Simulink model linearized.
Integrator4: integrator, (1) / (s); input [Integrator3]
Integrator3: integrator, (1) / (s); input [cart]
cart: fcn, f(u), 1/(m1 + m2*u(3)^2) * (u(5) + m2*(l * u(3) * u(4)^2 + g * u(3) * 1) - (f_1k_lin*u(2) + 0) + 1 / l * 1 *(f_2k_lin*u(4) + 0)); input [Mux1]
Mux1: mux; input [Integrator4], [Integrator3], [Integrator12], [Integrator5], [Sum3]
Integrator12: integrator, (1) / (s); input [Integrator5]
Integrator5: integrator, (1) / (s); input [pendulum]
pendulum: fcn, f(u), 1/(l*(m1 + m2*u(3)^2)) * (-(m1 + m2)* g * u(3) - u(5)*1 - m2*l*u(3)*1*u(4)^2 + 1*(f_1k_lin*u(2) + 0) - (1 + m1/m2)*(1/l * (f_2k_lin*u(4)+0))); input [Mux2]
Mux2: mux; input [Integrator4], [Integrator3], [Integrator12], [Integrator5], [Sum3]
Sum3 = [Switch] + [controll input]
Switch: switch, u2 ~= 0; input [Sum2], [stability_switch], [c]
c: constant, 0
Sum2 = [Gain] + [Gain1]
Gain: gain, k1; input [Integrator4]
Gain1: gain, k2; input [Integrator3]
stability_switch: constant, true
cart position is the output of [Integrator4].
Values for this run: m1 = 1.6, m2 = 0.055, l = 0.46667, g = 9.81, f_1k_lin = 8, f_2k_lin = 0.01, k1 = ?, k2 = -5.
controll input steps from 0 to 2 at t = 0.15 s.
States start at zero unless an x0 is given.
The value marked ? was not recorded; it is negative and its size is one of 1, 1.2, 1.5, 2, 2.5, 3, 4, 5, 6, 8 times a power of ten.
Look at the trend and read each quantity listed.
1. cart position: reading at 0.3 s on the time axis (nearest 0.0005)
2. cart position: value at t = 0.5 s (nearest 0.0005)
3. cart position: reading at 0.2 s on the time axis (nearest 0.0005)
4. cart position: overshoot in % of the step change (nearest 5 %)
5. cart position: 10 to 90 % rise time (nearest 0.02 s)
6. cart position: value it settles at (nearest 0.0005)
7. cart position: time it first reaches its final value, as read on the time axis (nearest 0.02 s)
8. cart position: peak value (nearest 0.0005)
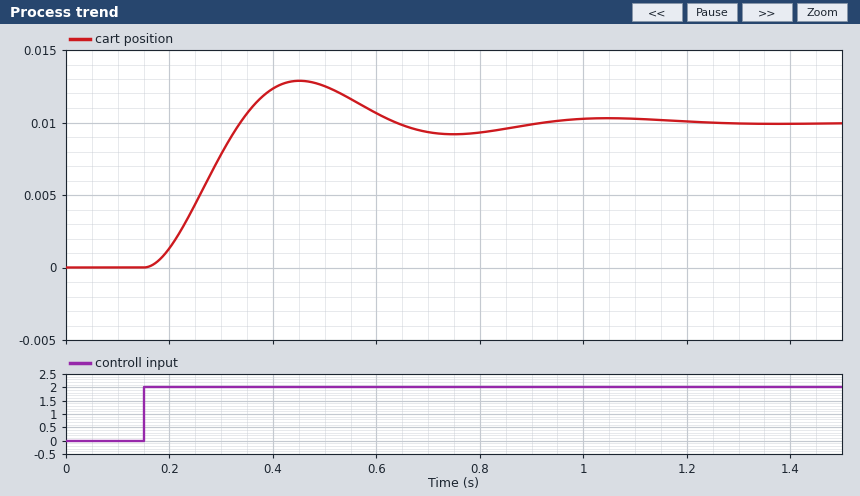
0.0080
0.0125
0.0015
30 %
0.12 s
0.0100
0.34 s
0.0130
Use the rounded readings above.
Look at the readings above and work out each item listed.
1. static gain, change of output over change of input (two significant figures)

0.0050
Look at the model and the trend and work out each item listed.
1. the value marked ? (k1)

-200
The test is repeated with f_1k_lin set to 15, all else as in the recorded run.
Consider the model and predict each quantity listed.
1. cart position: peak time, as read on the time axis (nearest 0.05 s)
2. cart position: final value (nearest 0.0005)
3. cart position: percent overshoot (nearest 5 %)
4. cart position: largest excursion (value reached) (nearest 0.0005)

0.50 s
0.0100
10 %
0.0110
